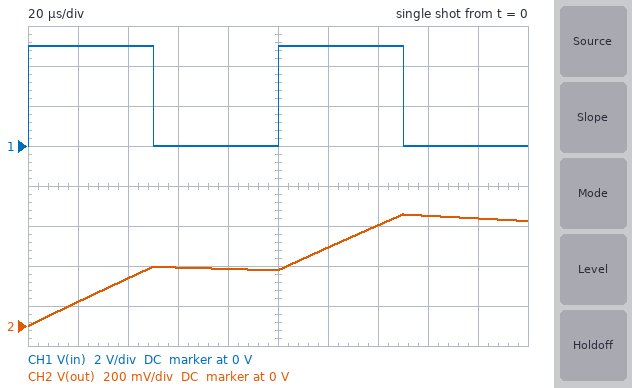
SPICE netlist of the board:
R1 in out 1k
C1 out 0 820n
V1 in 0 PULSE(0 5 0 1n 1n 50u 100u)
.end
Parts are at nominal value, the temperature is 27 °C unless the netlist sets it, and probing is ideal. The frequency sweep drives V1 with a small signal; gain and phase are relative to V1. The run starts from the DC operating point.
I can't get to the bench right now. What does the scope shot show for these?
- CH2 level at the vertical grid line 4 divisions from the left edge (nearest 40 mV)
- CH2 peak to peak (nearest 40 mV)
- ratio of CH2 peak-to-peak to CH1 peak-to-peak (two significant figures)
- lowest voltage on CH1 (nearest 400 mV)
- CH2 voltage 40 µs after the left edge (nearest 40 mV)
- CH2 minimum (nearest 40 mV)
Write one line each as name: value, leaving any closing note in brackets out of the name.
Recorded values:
CH2 level at the vertical grid line 4 divisions from the left edge: 280 mV
CH2 peak to peak: 560 mV
ratio of CH2 peak-to-peak to CH1 peak-to-peak: 0.11
lowest voltage on CH1: 0 V
CH2 voltage 40 µs after the left edge: 240 mV
CH2 minimum: 0 V
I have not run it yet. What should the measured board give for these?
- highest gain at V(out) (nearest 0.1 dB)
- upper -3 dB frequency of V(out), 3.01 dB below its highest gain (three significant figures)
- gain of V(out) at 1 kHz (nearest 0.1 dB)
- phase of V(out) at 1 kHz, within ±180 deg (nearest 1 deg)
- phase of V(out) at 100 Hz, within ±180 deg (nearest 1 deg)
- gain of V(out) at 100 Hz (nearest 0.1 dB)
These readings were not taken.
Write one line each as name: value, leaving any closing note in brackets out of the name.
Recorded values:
highest gain at V(out): 0 dB
upper -3 dB frequency of V(out), 3.01 dB below its highest gain: 194 Hz
gain of V(out) at 1 kHz: -14.4 dB
phase of V(out) at 1 kHz, within ±180 deg: -79 deg
phase of V(out) at 100 Hz, within ±180 deg: -27 deg
gain of V(out) at 100 Hz: -1.0 dB
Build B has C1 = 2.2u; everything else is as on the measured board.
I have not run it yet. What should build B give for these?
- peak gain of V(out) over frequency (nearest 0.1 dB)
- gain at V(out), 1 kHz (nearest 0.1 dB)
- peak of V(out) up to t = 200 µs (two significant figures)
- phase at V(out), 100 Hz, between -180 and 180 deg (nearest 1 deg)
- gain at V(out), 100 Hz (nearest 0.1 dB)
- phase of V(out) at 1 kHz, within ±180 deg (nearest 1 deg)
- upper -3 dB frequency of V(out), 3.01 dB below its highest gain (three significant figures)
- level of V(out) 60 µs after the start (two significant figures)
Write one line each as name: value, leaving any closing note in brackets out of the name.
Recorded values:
peak gain of V(out) over frequency: 0 dB
gain at V(out), 1 kHz: -22.8 dB
peak of V(out) up to t = 200 µs: 220 mV
phase at V(out), 100 Hz, between -180 and 180 deg: -54 deg
gain at V(out), 100 Hz: -4.6 dB
phase of V(out) at 1 kHz, within ±180 deg: -86 deg
upper -3 dB frequency of V(out), 3.01 dB below its highest gain: 72.3 Hz
level of V(out) 60 µs after the start: 110 mV
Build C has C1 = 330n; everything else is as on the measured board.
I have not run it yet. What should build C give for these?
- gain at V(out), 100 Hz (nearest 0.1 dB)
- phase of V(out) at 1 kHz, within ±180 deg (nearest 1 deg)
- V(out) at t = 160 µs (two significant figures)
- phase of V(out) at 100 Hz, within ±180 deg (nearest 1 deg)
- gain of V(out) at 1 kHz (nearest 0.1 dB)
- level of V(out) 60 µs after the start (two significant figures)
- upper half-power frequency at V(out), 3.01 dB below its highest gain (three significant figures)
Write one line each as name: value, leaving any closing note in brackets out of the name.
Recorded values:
gain at V(out), 100 Hz: -0.2 dB
phase of V(out) at 1 kHz, within ±180 deg: -64 deg
V(out) at t = 160 µs: 1.2 V
phase of V(out) at 100 Hz, within ±180 deg: -12 deg
gain of V(out) at 1 kHz: -7.2 dB
level of V(out) 60 µs after the start: 680 mV
upper half-power frequency at V(out), 3.01 dB below its highest gain: 482 Hz
